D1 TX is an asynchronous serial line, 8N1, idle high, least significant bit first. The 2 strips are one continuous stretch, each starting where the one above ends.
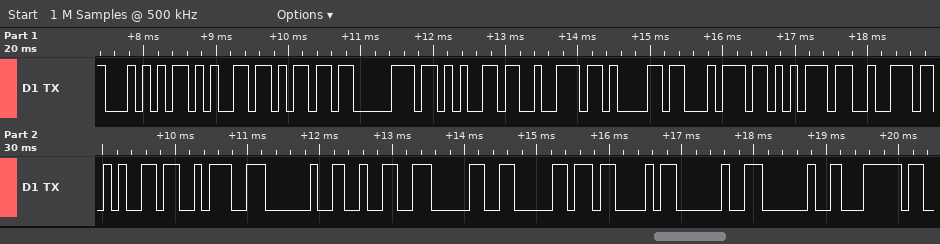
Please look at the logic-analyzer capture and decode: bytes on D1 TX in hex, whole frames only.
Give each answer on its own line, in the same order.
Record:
54 65 6D 70 65 72 61 74 75 72 65 3A 20 32 30 B0 43 20 20 7C
